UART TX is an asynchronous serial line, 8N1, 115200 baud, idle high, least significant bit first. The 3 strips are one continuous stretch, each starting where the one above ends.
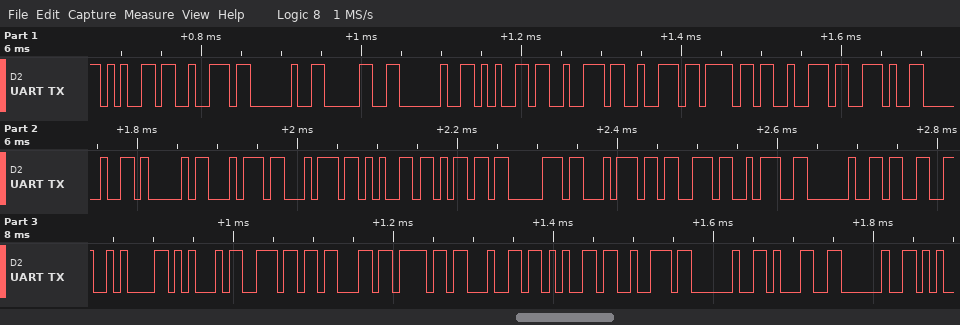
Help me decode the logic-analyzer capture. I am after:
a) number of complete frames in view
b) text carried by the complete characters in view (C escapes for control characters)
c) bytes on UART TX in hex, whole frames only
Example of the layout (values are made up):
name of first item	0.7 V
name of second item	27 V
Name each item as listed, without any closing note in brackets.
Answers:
number of complete frames in view	34
text carried by the complete characters in view	"er 0 error. Attempts: 3\nEncoder 1 "
bytes on UART TX in hex, whole frames only	0x65 0x72 0x20 0x30 0x20 0x65 0x72 0x72 0x6F 0x72 0x2E 0x20 0x41 0x74 0x74 0x65 0x6D 0x70 0x74 0x73 0x3A 0x20 0x33 0x0A 0x45 0x6E 0x63 0x6F 0x64 0x65 0x72 0x20 0x31 0x20
